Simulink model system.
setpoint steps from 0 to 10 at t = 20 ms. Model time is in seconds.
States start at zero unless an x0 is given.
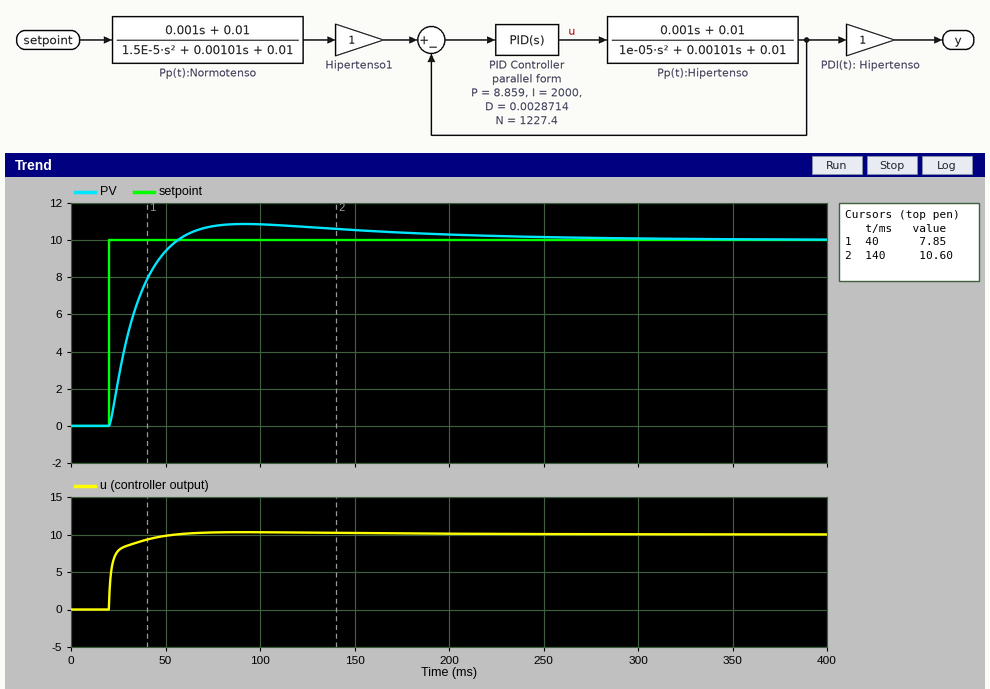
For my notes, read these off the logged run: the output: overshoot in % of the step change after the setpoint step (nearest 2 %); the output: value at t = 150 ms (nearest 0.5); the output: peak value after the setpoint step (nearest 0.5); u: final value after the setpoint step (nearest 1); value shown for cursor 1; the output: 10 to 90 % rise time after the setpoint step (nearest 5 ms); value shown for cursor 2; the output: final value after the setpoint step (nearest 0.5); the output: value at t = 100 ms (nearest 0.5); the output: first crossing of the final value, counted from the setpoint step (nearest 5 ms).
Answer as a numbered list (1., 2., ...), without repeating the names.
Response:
1. 8 %
2. 10.5
3. 11.0
4. 10
5. 7.85
6. 25 ms
7. 10.60
8. 10.0
9. 11.0
10. 35 ms
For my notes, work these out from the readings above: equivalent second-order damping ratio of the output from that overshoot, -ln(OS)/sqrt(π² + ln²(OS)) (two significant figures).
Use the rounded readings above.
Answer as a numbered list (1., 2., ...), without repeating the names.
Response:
1. 0.63
